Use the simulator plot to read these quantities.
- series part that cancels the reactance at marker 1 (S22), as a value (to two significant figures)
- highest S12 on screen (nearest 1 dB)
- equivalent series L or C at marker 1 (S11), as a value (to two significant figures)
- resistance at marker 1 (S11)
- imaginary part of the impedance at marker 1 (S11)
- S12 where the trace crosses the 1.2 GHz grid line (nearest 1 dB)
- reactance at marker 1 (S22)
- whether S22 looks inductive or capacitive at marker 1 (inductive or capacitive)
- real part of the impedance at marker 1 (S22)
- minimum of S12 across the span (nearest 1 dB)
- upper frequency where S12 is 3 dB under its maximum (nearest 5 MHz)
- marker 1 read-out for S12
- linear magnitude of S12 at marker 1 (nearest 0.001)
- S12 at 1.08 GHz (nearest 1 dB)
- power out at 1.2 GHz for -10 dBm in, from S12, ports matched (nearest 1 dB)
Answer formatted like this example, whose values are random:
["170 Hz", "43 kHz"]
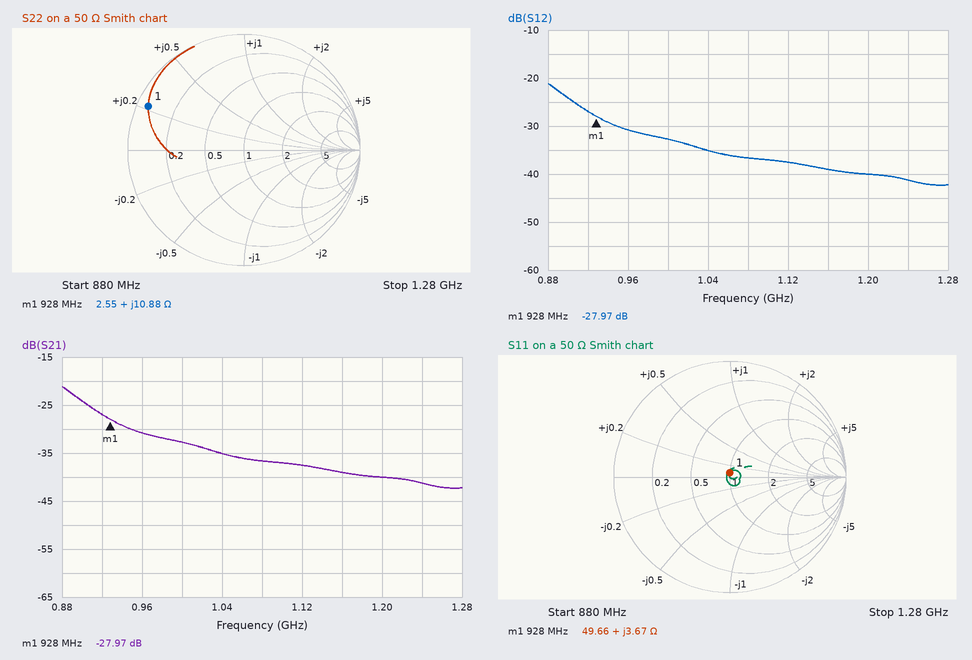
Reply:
["16 pF", "-21 dB", "630 pH", "49.66 Ω", "+3.67 Ω", "-40 dB", "+10.88 Ω", "inductive", "2.55 Ω", "-42 dB", "900 MHz", "-27.97 dB", "0.040", "-37 dB", "-50 dBm"]
